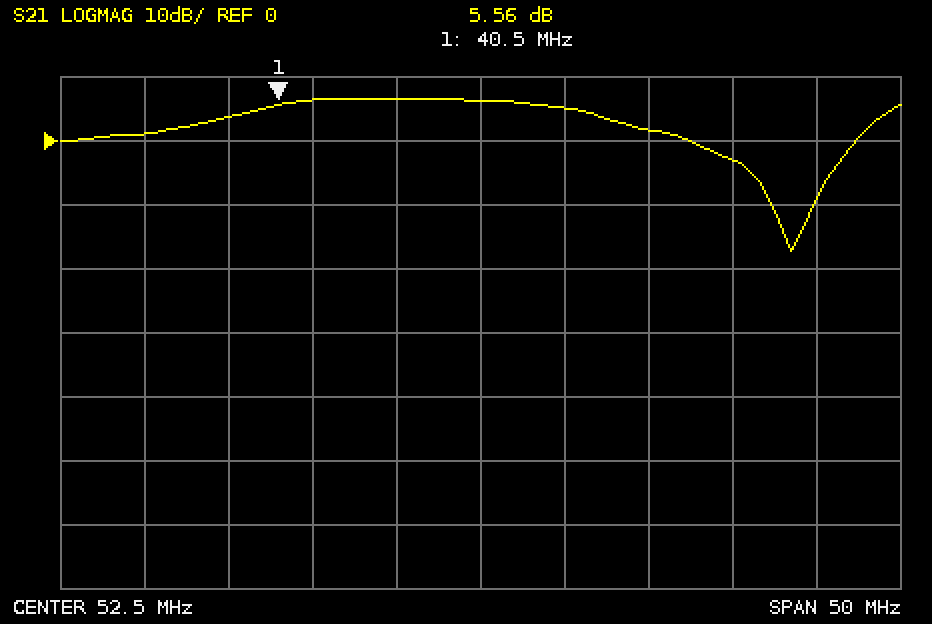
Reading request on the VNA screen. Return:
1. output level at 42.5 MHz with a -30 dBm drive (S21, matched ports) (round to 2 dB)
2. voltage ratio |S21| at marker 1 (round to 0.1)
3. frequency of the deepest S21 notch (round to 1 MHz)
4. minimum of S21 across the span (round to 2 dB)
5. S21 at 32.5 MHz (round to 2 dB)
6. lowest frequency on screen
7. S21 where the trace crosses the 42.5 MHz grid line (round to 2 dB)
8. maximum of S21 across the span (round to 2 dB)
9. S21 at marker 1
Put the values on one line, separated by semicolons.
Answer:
-24 dBm; 1.9; 71 MHz; -18 dB; 2 dB; 27.5 MHz; 6 dB; 6 dB; 5.56 dB
